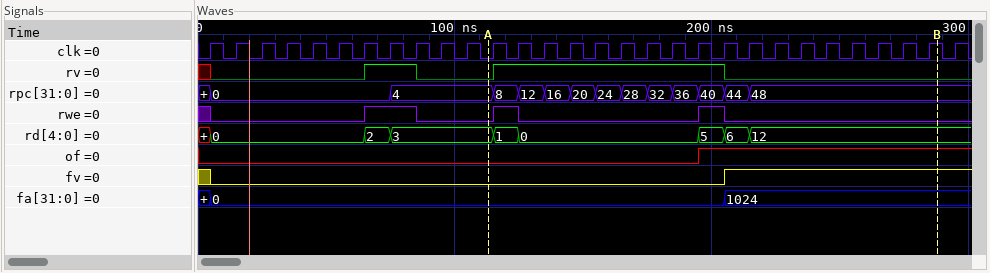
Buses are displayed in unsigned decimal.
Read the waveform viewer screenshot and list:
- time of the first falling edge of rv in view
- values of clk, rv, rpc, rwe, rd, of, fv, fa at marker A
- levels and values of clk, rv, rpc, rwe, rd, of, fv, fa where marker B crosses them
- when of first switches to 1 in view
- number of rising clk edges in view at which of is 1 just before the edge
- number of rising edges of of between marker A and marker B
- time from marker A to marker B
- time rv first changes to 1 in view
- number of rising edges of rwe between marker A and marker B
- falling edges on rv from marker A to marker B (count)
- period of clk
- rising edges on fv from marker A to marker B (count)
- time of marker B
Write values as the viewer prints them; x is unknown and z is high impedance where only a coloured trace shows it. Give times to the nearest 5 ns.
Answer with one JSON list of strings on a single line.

["85 ns", "clk=0, rv=0, rpc=4, rwe=0, rd=3, of=0, fv=0, fa=0", "clk=1, rv=0, rpc=48, rwe=0, rd=12, of=1, fv=1, fa=1024", "195 ns", "10", "1", "175 ns", "65 ns", "2", "1", "10 ns", "1", "290 ns"]
